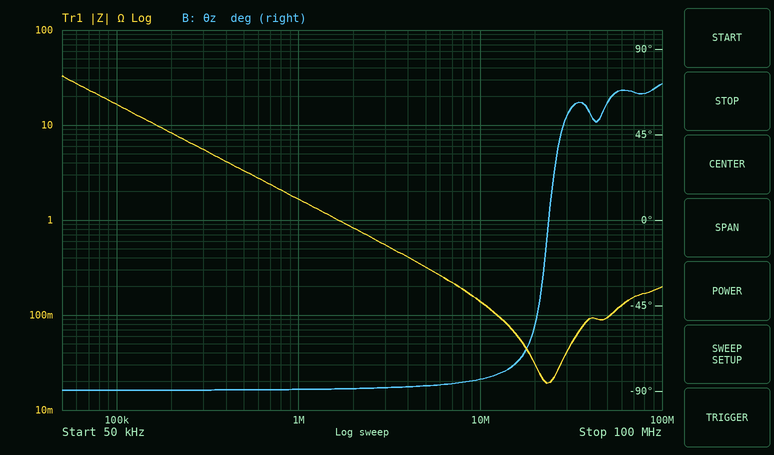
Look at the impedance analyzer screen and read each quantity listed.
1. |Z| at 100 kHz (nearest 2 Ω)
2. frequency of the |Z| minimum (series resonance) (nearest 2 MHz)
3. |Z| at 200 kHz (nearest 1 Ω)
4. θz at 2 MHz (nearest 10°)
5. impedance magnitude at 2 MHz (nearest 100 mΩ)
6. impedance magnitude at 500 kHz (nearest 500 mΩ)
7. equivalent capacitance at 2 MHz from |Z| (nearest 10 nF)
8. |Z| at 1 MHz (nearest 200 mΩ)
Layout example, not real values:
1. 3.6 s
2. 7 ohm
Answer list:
1. 16 Ω
2. 24 MHz
3. 8 Ω
4. -90°
5. 800 mΩ
6. 3.5 Ω
7. 100 nF
8. 1.6 Ω
